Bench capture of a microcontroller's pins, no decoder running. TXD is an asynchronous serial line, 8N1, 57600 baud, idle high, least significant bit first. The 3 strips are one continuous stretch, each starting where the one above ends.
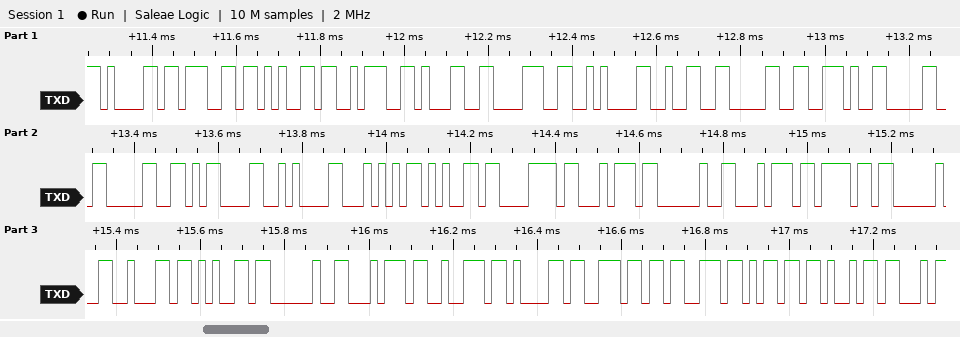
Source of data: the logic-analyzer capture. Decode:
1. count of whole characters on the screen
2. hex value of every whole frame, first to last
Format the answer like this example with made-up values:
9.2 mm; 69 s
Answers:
32; 61 67 65 3A 31 38 0A 32 30 2E 30 30 0D 0A 54 65 78 74 20 74 6F 20 62 65 20 74 72 61 6E 73 6D 69
